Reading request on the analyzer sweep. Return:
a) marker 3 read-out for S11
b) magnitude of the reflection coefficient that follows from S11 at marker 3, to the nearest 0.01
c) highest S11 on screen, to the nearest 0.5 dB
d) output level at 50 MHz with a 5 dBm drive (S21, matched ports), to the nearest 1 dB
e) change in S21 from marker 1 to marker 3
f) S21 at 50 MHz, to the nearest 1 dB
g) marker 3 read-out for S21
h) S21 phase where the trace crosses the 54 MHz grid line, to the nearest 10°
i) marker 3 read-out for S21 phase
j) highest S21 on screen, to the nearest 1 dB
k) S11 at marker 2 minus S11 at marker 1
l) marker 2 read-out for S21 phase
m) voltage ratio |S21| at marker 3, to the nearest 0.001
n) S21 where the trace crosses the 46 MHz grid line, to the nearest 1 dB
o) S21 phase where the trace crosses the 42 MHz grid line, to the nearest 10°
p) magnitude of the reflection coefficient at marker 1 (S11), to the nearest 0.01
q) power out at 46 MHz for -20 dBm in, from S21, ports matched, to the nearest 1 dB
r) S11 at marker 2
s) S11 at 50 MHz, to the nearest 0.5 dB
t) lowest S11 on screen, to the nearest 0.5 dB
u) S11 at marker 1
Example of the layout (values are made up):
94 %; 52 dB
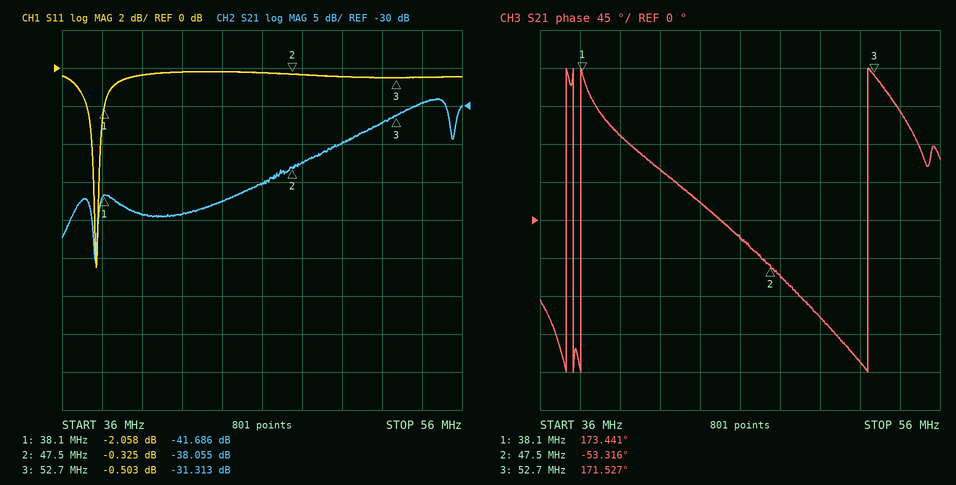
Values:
-0.503 dB; 0.94; 0.0 dB; -30 dBm; 10.373 dB; -35 dB; -31.313 dB; 130°; 171.527°; -29 dB; 1.733 dB; -53.316°; 0.027; -40 dB; 60°; 0.79; -60 dBm; -0.325 dB; -0.5 dB; -10.5 dB; -2.058 dB
